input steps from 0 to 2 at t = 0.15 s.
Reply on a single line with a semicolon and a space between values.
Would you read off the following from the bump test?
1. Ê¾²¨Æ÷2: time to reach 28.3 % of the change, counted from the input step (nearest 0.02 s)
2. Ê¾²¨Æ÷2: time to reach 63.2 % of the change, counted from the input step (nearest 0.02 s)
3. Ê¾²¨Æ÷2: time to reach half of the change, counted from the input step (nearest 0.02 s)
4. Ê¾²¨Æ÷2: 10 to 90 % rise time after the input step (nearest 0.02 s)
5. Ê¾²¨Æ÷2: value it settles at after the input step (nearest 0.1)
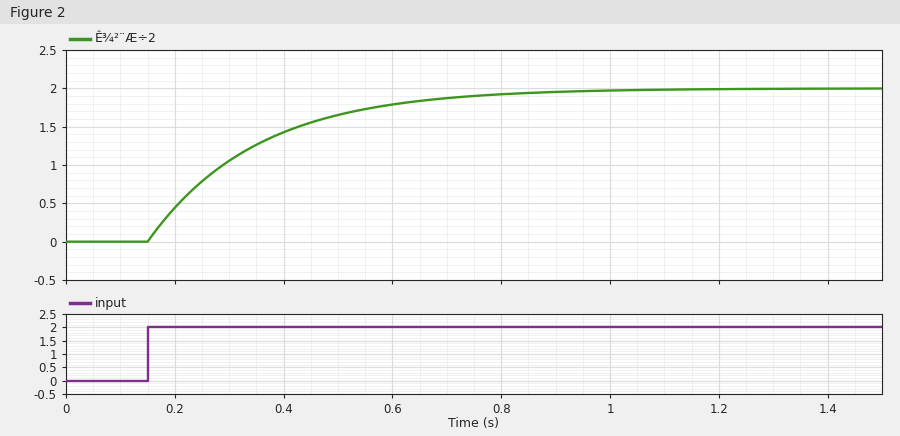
0.06 s; 0.20 s; 0.14 s; 0.44 s; 2.0
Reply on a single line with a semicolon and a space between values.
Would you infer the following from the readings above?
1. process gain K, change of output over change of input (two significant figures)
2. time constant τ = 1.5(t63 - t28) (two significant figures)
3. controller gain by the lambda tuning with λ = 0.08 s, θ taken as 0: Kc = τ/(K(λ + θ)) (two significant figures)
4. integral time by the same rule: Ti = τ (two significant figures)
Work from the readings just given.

1.0; 0.21 s; 2.6; 0.21 s
